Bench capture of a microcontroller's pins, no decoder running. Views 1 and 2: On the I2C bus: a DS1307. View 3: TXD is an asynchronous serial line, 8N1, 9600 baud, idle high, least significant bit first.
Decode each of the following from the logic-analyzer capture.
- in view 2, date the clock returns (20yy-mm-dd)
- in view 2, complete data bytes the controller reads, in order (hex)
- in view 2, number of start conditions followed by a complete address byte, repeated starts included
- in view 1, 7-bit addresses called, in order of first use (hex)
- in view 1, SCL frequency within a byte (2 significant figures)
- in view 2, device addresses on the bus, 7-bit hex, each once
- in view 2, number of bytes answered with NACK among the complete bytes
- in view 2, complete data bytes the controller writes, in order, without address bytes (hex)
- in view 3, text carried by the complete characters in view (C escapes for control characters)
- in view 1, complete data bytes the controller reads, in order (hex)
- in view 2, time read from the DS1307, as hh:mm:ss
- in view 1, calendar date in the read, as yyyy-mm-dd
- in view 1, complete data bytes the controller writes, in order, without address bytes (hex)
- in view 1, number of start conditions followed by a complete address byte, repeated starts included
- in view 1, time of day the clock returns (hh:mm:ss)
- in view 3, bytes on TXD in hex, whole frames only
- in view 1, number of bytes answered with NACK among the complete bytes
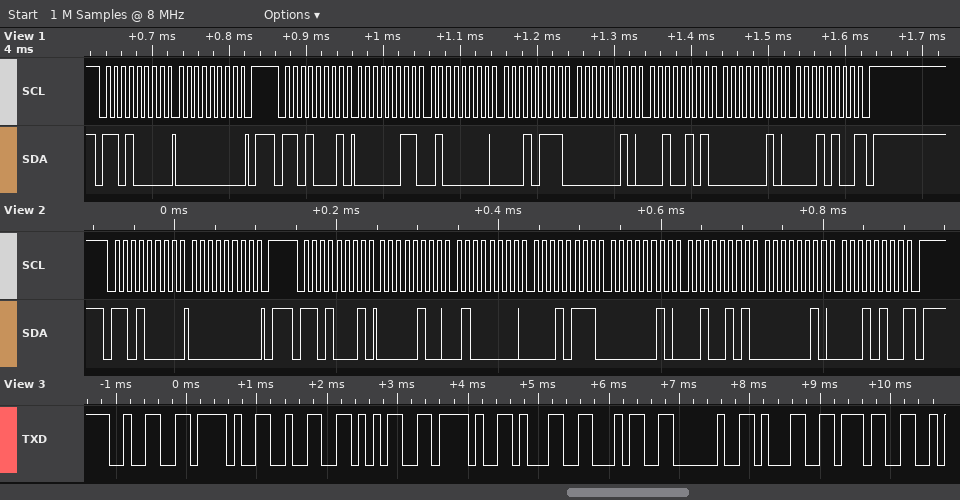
2014-02-25
04 40 17 02 25 02 14
2
0x68
100 kHz
0x68
1
00
"2/25/14 17"
03 40 17 02 25 02 14
17:40:04
2014-02-25
00
2
17:40:03
32 2F 32 35 2F 31 34 20 31 37
1
